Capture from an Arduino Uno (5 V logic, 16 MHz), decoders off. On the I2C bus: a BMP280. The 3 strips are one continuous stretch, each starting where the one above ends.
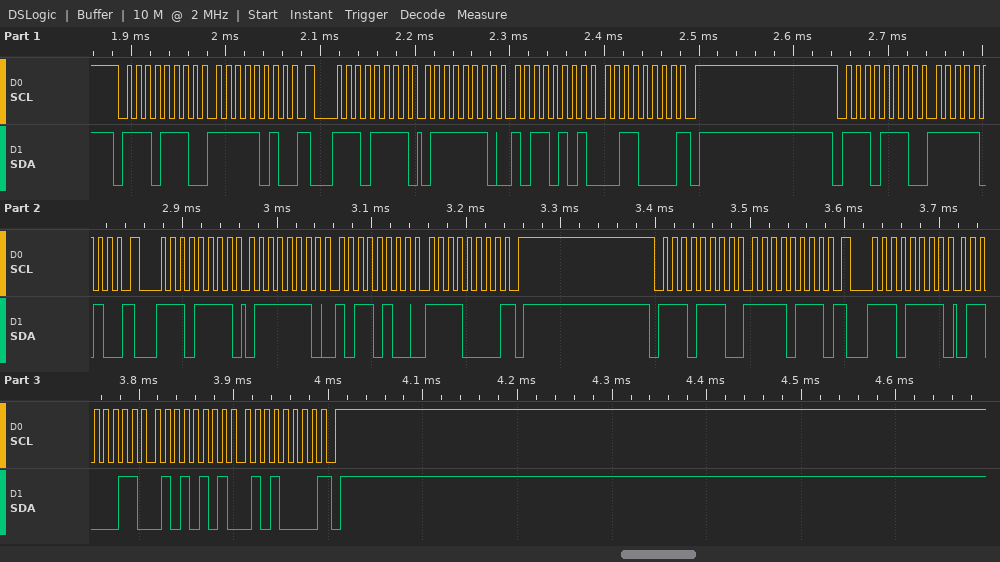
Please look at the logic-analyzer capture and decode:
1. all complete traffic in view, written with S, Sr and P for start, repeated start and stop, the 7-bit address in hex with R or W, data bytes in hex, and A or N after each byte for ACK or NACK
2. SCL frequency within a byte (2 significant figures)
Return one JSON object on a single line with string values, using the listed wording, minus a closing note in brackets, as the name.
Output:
{"all complete traffic in view, written with S, Sr and P for start, repeated start and stop, the 7-bit address in hex with R or W, data bytes in hex, and A or N after each byte for ACK or NACK": "S 77W A FA A Sr 77R A 7E A B5 A 30 N P S 77W A FA A Sr 77R A 7E A B4 A F0 N P S 77W A F7 A Sr 77R A 63 A 55 A 50 N P", "SCL frequency within a byte": "100 kHz"}
